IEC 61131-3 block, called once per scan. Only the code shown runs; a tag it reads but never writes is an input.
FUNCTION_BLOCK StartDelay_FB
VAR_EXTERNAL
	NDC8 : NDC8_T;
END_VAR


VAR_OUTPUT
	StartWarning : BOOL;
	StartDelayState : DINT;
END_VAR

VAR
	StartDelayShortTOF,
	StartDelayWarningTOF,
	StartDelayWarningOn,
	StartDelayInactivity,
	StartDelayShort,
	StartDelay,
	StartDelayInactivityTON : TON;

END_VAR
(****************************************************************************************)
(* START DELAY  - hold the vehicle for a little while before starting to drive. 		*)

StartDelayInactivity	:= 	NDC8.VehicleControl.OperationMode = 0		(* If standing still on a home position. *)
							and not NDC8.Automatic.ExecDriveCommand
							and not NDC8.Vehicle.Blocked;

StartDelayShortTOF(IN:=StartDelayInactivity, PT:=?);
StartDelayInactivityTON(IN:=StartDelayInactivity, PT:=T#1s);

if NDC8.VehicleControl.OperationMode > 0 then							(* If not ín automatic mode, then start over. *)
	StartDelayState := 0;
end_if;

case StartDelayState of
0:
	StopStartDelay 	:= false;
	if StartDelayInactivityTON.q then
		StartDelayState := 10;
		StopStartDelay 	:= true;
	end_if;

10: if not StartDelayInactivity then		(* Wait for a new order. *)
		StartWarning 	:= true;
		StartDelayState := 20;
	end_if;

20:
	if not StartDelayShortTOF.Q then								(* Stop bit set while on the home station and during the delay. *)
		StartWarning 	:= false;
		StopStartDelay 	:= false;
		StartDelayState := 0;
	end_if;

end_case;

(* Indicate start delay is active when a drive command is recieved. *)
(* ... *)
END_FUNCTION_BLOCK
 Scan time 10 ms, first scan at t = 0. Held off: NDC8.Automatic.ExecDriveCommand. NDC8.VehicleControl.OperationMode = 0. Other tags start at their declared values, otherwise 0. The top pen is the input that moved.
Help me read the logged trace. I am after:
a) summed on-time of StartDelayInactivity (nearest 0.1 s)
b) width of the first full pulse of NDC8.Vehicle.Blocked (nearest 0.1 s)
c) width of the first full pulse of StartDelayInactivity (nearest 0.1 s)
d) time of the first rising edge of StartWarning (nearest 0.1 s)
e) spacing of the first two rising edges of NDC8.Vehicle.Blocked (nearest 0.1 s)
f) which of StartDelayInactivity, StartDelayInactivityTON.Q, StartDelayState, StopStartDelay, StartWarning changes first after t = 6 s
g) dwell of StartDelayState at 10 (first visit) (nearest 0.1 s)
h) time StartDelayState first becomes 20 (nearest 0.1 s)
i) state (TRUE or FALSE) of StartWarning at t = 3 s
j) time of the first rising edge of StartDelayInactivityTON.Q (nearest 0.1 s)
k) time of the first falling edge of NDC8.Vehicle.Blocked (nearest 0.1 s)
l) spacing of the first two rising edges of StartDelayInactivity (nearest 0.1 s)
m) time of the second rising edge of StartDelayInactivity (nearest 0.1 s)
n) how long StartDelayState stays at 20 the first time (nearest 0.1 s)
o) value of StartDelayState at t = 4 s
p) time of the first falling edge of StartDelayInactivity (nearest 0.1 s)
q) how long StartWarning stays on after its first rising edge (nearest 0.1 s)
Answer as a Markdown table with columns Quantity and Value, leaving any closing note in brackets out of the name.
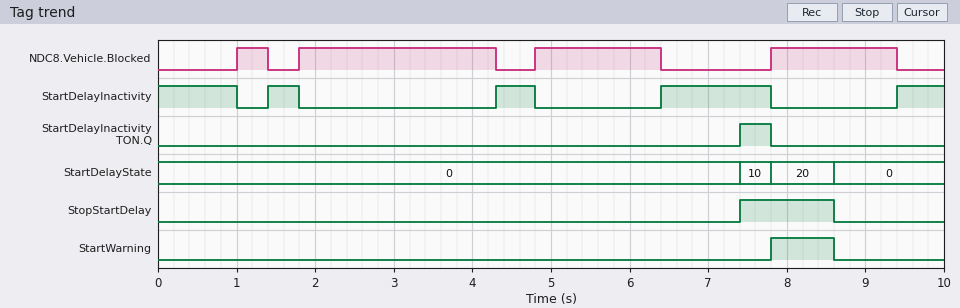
| Quantity | Value |
|---|---|
| summed on-time of StartDelayInactivity | 3.9 s |
| width of the first full pulse of NDC8.Vehicle.Blocked | 0.4 s |
| width of the first full pulse of StartDelayInactivity | 0.4 s |
| time of the first rising edge of StartWarning | 7.8 s |
| spacing of the first two rising edges of NDC8.Vehicle.Blocked | 0.8 s |
| which of StartDelayInactivity, StartDelayInactivityTON.Q, StartDelayState, StopStartDelay, StartWarning changes first after t = 6 s | StartDelayInactivity |
| dwell of StartDelayState at 10 (first visit) | 0.4 s |
| time StartDelayState first becomes 20 | 7.8 s |
| state (TRUE or FALSE) of StartWarning at t = 3 s | FALSE |
| time of the first rising edge of StartDelayInactivityTON.Q | 7.4 s |
| time of the first falling edge of NDC8.Vehicle.Blocked | 1.4 s |
| spacing of the first two rising edges of StartDelayInactivity | 2.9 s |
| time of the second rising edge of StartDelayInactivity | 4.3 s |
| how long StartDelayState stays at 20 the first time | 0.8 s |
| value of StartDelayState at t = 4 s | 0 |
| time of the first falling edge of StartDelayInactivity | 1.0 s |
| how long StartWarning stays on after its first rising edge | 0.8 s |
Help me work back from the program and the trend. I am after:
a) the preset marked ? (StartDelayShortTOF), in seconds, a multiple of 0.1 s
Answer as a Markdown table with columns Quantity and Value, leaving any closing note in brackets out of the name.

| Quantity | Value |
|---|---|
| the preset marked ? (StartDelayShortTOF), in seconds, a multiple of 0.1 s | 0.8 s |
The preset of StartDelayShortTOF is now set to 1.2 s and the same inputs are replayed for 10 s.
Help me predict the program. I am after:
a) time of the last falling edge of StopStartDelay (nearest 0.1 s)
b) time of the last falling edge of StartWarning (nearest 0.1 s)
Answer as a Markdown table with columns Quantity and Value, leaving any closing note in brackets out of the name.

| Quantity | Value |
|---|---|
| time of the last falling edge of StopStartDelay | 9.0 s |
| time of the last falling edge of StartWarning | 9.0 s |
